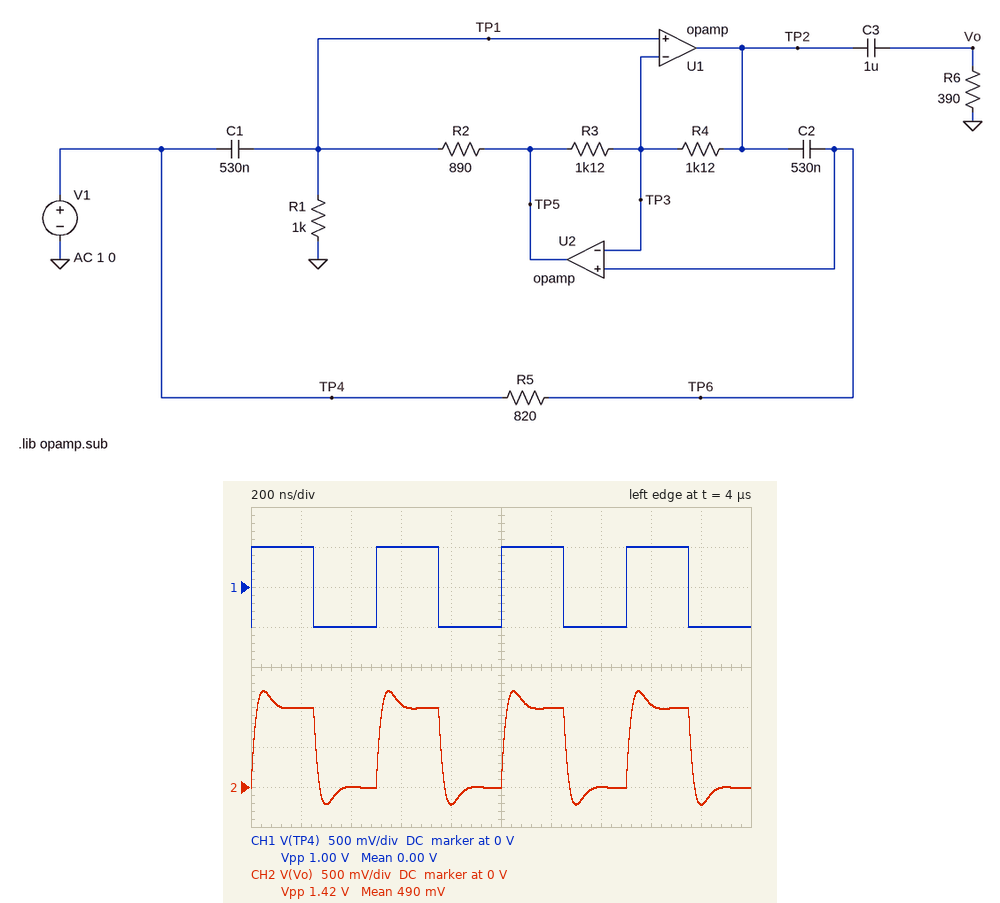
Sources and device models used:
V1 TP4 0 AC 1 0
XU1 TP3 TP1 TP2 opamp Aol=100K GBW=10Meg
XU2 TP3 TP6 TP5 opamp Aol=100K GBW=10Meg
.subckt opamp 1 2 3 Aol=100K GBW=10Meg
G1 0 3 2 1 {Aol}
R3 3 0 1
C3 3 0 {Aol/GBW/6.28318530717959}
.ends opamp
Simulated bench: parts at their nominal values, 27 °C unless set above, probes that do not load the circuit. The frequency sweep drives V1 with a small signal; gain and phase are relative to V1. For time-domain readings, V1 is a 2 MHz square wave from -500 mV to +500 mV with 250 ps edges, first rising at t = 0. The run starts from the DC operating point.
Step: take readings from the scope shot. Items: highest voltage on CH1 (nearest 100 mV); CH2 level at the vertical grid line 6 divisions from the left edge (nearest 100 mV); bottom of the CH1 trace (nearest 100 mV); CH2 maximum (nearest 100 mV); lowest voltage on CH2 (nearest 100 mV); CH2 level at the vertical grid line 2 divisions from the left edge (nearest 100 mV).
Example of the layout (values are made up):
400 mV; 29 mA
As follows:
500 mV; 1.0 V; -500 mV; 1.2 V; -200 mV; 0 V
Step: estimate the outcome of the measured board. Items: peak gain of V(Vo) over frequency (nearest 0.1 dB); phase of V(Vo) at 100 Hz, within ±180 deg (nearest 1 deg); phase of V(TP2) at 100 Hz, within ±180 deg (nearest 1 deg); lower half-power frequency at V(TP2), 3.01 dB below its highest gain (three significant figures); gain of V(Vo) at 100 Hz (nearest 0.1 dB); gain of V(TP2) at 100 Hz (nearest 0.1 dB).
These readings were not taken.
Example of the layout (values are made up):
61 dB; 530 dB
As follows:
0 dB; 61 deg; -15 deg; 311 Hz; -42.8 dB; -30.3 dB
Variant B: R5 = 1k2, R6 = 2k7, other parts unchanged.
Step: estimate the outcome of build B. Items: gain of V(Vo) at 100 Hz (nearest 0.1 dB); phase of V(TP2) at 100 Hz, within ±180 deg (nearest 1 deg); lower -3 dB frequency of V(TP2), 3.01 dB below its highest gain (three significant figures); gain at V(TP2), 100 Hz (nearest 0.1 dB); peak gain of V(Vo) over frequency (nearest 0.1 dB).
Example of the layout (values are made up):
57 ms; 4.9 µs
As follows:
-42.3 dB; 158 deg; 267 Hz; -41.0 dB; 0.6 dB
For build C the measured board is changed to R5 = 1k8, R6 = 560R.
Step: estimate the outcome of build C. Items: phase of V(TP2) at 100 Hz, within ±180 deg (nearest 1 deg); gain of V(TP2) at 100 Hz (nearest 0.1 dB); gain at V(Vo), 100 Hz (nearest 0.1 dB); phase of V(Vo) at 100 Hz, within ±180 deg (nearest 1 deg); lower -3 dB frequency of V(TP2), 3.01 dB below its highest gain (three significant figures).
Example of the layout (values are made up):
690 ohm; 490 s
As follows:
147 deg; -23.2 dB; -32.8 dB; -142 deg; 239 Hz
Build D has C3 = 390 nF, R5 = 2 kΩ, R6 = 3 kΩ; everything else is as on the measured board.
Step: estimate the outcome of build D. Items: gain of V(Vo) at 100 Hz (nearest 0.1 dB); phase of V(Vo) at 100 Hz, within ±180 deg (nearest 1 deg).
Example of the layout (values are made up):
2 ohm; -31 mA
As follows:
-25.7 dB; -163 deg
